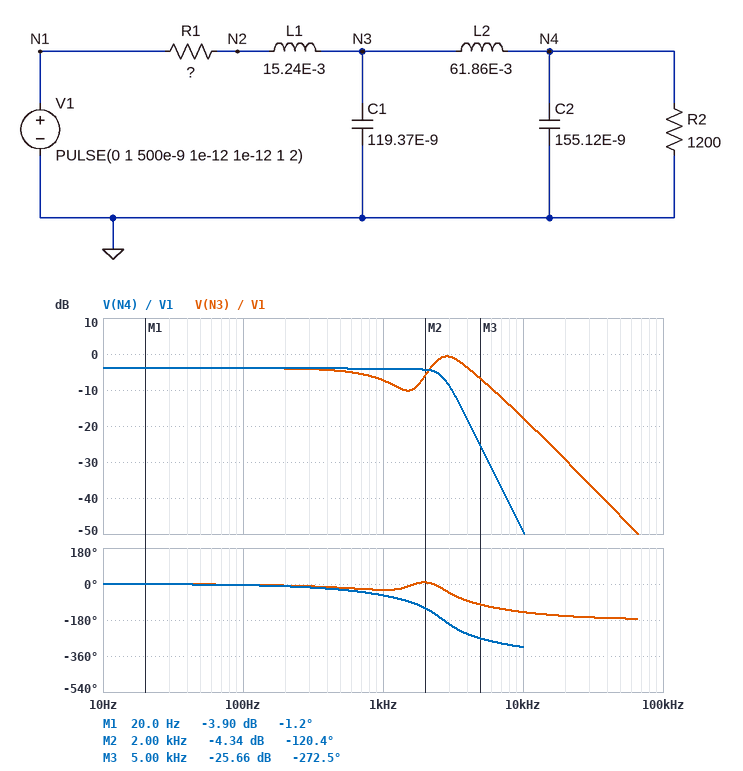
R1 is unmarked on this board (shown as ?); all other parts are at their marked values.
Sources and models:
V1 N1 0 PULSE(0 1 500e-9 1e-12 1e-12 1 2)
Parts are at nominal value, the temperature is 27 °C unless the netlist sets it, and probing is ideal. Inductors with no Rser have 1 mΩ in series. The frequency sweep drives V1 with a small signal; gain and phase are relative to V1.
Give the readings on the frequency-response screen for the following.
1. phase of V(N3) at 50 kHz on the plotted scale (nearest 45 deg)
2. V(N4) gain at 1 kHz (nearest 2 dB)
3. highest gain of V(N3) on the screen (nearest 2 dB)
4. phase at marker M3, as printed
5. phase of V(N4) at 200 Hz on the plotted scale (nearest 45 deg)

-180 deg
-4 dB
0 dB
-272.5 deg
0 deg
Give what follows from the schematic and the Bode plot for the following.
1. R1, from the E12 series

680 Ω
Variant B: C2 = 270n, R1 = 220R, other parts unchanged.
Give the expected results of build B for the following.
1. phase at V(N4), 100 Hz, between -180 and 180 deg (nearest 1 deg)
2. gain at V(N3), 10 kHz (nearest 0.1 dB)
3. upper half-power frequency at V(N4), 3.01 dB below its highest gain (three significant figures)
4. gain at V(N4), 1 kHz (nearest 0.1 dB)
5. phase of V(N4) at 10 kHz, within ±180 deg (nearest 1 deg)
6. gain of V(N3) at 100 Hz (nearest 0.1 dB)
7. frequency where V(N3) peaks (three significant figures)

-5 deg
-15.8 dB
1.51 kHz
1.3 dB
18 deg
-1.5 dB
3.91 kHz
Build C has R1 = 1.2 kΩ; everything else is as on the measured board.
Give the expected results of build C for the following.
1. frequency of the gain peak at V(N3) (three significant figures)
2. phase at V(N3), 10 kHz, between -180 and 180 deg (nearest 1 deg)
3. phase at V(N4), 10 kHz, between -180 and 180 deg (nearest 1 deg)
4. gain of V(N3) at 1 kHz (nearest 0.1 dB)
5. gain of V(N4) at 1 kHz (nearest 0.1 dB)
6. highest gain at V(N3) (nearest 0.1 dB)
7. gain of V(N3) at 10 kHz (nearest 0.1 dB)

2.62 kHz
-124 deg
61 deg
-10.8 dB
-7.7 dB
-2.6 dB
-20.4 dB
